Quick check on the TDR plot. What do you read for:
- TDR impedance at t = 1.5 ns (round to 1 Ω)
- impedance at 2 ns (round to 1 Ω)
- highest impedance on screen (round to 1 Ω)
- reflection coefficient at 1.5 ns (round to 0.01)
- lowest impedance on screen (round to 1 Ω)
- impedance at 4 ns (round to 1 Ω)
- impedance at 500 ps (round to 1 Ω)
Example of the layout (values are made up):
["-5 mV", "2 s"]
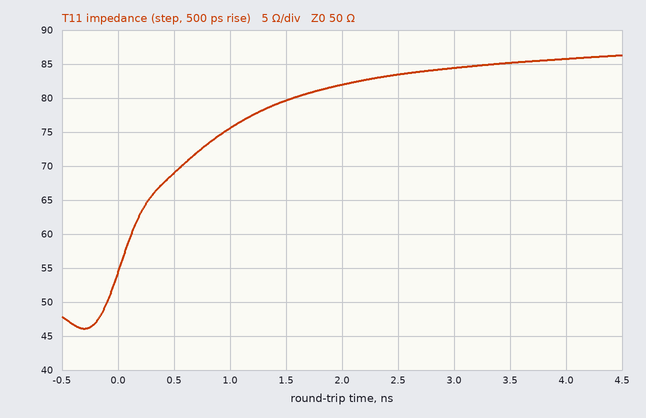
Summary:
["80 Ω", "82 Ω", "86 Ω", "+0.23", "46 Ω", "86 Ω", "69 Ω"]
